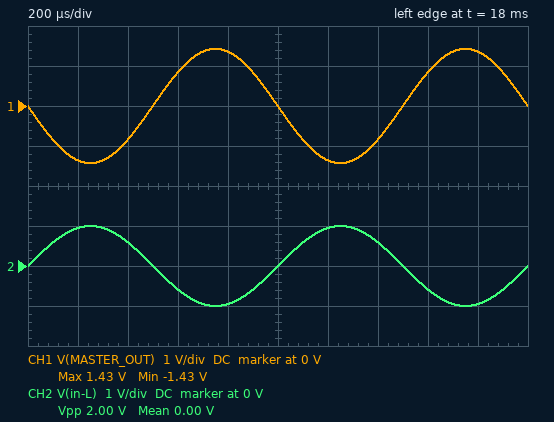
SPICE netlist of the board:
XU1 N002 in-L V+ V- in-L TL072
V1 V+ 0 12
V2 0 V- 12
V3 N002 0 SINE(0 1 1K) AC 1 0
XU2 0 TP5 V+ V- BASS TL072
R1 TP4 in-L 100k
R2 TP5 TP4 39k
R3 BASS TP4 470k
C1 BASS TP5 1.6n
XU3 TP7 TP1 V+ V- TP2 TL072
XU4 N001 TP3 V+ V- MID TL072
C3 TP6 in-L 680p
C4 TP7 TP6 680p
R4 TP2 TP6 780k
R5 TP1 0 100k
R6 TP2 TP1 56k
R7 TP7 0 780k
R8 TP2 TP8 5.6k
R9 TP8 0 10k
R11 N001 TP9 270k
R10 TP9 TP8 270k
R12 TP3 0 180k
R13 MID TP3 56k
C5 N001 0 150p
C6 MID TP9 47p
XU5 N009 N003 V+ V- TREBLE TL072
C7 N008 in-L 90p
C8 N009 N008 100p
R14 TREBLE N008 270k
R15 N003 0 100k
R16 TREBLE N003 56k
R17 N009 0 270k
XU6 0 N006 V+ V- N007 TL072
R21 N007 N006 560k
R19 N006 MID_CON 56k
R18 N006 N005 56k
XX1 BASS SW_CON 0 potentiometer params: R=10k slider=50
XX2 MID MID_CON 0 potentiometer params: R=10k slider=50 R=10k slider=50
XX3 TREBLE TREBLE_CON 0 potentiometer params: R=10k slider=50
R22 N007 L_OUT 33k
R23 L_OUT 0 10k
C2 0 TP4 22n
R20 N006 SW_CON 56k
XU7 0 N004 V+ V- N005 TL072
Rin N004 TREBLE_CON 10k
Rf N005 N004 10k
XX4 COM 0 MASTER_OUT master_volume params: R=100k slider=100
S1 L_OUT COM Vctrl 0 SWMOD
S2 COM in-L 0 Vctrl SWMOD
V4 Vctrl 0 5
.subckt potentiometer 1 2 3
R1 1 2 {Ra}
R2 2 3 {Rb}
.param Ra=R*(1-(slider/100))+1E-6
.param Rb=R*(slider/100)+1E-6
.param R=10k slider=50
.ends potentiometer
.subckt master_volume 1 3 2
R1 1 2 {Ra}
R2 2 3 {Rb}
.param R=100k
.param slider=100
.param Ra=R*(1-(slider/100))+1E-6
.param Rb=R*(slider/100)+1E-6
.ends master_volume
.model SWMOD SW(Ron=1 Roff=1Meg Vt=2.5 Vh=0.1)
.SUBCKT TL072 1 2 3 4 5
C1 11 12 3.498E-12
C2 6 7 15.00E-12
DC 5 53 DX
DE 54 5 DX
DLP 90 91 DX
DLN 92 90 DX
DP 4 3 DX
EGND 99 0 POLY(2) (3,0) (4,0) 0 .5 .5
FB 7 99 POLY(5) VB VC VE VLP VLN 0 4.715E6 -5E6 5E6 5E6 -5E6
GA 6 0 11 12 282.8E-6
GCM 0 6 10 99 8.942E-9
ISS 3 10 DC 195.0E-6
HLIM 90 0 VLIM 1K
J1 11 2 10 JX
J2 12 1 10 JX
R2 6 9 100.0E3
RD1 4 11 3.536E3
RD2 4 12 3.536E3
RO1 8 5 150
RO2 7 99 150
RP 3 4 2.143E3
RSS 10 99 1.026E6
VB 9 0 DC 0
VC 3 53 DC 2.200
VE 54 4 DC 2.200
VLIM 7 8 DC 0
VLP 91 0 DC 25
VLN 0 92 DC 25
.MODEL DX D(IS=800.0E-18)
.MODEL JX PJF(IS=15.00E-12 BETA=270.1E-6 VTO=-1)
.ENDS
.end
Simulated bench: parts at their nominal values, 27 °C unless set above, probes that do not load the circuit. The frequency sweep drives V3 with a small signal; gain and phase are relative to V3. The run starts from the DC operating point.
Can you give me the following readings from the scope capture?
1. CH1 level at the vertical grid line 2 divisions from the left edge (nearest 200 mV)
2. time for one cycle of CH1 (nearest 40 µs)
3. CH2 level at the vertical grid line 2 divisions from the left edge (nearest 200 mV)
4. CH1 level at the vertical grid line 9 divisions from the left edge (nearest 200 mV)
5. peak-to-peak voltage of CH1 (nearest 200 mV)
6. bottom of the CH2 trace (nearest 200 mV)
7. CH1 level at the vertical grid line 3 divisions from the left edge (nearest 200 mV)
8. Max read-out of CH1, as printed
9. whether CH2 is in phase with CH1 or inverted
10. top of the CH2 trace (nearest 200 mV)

-800 mV
1.00 ms
600 mV
1.4 V
2.8 V
-1.0 V
800 mV
1.43 V
inverted
1.0 V
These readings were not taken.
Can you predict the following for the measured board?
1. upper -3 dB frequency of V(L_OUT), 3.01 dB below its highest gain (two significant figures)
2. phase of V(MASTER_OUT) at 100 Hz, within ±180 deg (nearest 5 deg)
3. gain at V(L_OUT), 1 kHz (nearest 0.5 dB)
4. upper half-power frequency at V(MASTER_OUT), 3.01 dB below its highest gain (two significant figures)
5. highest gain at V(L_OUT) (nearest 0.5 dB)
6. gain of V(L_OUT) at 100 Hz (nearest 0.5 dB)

240 Hz
-35 deg
4.0 dB
200 Hz
14.5 dB
14.5 dB
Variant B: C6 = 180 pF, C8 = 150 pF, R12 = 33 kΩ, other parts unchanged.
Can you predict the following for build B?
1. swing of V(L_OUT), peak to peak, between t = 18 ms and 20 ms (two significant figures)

4.5 V
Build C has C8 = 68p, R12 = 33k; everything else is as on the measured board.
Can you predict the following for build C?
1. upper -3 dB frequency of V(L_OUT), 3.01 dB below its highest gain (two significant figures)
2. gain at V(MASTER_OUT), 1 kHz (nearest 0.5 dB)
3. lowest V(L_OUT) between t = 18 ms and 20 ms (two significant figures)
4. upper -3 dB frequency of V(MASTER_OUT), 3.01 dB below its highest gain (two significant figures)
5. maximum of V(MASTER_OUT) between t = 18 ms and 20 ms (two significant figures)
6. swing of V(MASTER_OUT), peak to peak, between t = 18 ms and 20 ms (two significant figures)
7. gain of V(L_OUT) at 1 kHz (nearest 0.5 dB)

370 Hz
-15.5 dB
-2.2 V
240 Hz
2.2 V
4.5 V
9.5 dB
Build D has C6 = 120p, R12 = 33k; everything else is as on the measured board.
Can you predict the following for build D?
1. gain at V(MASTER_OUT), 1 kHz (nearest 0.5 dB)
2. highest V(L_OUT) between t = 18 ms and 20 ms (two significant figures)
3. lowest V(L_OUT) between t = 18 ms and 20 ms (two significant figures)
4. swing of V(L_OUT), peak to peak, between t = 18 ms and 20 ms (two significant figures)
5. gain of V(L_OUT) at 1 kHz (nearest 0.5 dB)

-14.0 dB
2.2 V
-2.2 V
4.5 V
10.5 dB
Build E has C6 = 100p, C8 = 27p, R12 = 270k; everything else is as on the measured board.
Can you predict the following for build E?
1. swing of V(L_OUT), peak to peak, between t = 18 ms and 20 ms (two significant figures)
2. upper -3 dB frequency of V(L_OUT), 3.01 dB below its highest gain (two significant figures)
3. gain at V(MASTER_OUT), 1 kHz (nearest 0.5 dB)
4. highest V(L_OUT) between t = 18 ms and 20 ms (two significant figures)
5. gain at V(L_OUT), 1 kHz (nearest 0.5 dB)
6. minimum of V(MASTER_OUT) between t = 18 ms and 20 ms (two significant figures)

2.7 V
230 Hz
-28.5 dB
1.3 V
3.0 dB
-1.3 V
